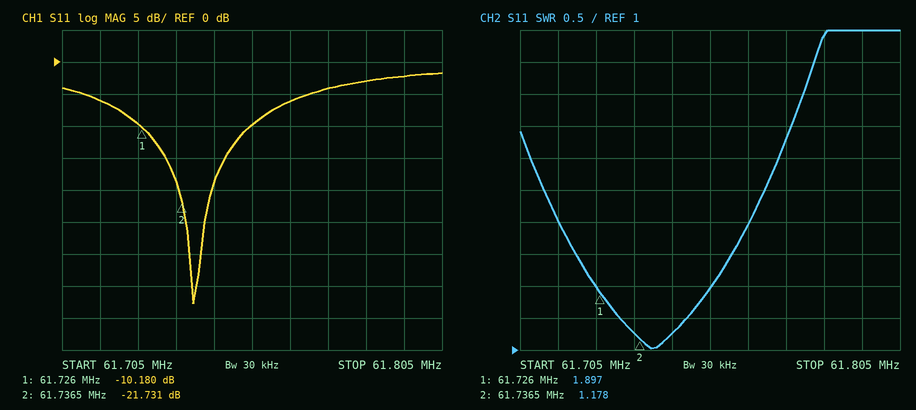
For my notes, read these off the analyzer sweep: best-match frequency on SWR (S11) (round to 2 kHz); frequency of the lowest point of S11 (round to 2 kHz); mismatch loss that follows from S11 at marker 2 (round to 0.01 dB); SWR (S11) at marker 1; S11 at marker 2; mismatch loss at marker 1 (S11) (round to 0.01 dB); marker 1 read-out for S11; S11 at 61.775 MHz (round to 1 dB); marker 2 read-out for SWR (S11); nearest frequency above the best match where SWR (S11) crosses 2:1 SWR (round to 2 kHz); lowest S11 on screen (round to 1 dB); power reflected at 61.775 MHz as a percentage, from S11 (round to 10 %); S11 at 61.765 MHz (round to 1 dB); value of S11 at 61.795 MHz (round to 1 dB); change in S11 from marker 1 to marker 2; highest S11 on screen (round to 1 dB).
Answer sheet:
61.740 MHz
61.740 MHz
0.03 dB
1.897
-21.731 dB
0.44 dB
-10.180 dB
-4 dB
1.178
61.756 MHz
-38 dB
40 %
-6 dB
-2 dB
-11.551 dB
-2 dB
